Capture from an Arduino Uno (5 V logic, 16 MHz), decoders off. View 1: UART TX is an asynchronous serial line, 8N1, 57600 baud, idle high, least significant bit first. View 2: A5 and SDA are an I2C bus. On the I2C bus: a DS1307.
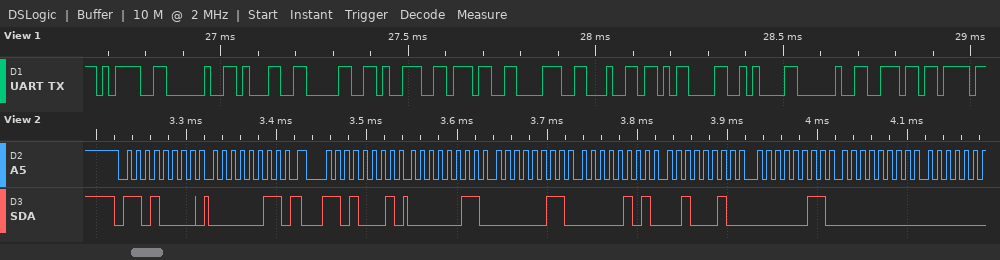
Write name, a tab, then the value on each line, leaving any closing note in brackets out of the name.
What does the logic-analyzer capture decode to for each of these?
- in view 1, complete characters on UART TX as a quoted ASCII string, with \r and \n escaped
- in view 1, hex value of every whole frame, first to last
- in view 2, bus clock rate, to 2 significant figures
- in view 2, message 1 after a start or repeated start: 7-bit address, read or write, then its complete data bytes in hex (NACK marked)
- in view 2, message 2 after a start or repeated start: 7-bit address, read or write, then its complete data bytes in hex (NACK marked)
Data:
in view 1, complete characters on UART TX as a quoted ASCII string, with \r and \n escaped	"= 10978d\r\n n"
in view 1, hex value of every whole frame, first to last	3D 20 31 30 39 37 38 64 0D 0A 20 6E
in view 2, bus clock rate, to 2 significant figures	100 kHz
in view 2, message 1 after a start or repeated start: 7-bit address, read or write, then its complete data bytes in hex	0x68 write: 03
in view 2, message 2 after a start or repeated start: 7-bit address, read or write, then its complete data bytes in hex	0x68 read: 03 03 05 22 03 00
